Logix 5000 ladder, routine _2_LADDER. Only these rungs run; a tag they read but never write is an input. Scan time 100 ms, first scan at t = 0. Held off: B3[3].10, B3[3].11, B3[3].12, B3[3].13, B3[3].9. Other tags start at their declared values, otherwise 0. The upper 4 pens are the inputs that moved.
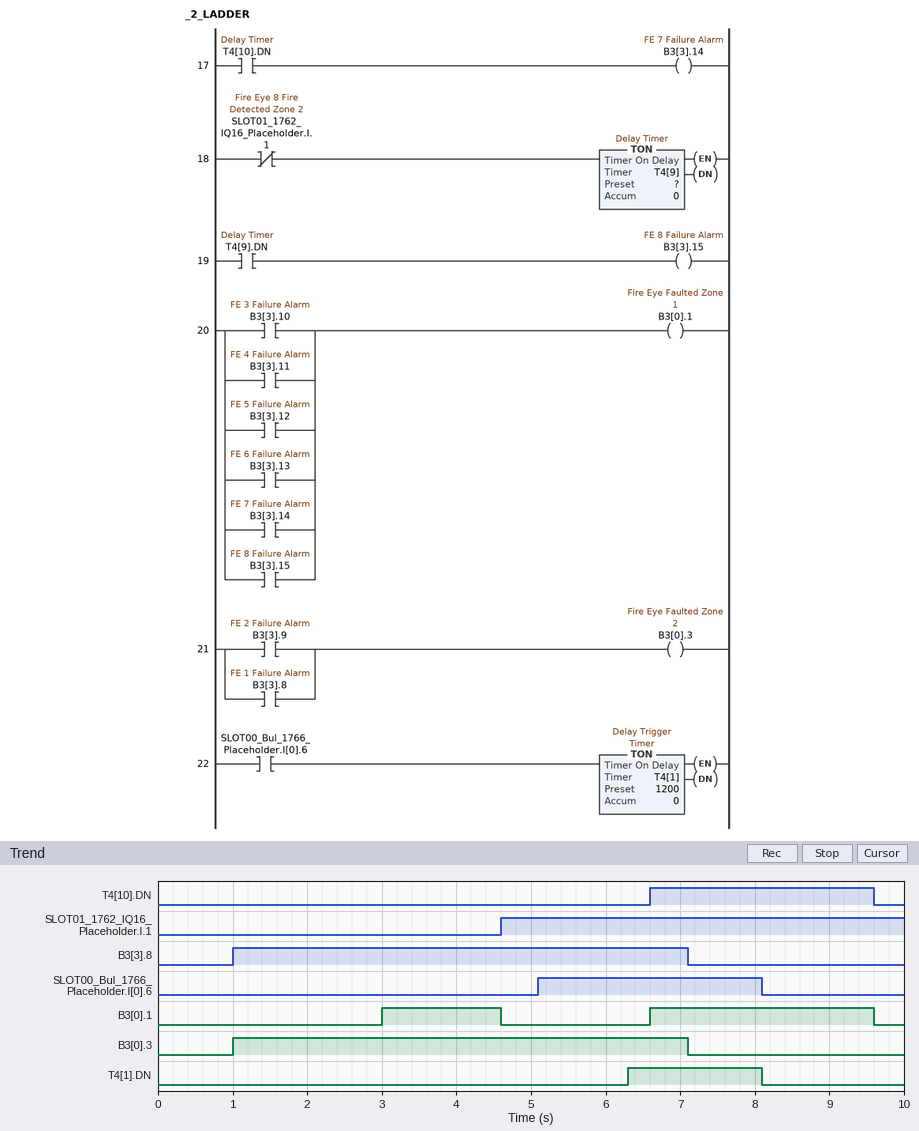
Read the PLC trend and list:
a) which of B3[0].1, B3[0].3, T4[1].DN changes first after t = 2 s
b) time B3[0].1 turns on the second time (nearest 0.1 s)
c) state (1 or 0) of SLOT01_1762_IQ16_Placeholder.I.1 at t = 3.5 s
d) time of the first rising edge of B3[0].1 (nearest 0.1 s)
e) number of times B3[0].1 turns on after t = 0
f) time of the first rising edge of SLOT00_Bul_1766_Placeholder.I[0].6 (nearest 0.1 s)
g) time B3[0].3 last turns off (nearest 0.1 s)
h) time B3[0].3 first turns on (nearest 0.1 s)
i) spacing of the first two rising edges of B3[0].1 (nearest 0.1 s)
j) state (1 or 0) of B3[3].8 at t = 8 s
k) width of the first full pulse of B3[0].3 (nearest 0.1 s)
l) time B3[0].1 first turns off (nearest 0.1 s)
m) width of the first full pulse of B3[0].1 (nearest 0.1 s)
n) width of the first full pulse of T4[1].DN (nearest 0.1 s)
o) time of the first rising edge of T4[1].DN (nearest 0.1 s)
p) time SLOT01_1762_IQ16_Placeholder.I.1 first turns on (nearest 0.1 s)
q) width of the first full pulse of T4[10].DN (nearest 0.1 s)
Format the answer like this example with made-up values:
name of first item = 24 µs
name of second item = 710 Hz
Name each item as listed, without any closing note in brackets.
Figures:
which of B3[0].1, B3[0].3, T4[1].DN changes first after t = 2 s = B3[0].1
time B3[0].1 turns on the second time = 6.6 s
state (1 or 0) of SLOT01_1762_IQ16_Placeholder.I.1 at t = 3.5 s = 0
time of the first rising edge of B3[0].1 = 3.0 s
number of times B3[0].1 turns on after t = 0 = 2
time of the first rising edge of SLOT00_Bul_1766_Placeholder.I[0].6 = 5.1 s
time B3[0].3 last turns off = 7.1 s
time B3[0].3 first turns on = 1.0 s
spacing of the first two rising edges of B3[0].1 = 3.6 s
state (1 or 0) of B3[3].8 at t = 8 s = 0
width of the first full pulse of B3[0].3 = 6.1 s
time B3[0].1 first turns off = 4.6 s
width of the first full pulse of B3[0].1 = 1.6 s
width of the first full pulse of T4[1].DN = 1.8 s
time of the first rising edge of T4[1].DN = 6.3 s
time SLOT01_1762_IQ16_Placeholder.I.1 first turns on = 4.6 s
width of the first full pulse of T4[10].DN = 3.0 s
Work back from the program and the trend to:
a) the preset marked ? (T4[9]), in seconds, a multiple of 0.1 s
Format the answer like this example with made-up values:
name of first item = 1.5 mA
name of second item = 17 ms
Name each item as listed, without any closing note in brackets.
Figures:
the preset marked ? (T4[9]), in seconds, a multiple of 0.1 s = 3.0 s
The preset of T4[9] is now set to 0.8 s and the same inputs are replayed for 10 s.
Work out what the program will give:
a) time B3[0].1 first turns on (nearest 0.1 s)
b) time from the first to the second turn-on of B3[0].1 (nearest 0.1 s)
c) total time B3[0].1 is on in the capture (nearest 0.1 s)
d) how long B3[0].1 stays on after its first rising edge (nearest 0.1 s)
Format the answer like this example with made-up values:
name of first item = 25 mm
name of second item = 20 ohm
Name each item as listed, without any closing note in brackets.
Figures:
time B3[0].1 first turns on = 0.8 s
time from the first to the second turn-on of B3[0].1 = 5.8 s
total time B3[0].1 is on in the capture = 6.8 s
how long B3[0].1 stays on after its first rising edge = 3.8 s
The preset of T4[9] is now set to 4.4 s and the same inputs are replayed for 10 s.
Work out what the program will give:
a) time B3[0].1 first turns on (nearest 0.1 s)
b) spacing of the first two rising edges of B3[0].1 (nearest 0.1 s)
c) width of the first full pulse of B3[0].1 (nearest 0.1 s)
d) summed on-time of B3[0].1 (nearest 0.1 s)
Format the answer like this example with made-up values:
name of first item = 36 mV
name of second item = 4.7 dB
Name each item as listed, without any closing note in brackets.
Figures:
time B3[0].1 first turns on = 4.4 s
spacing of the first two rising edges of B3[0].1 = 2.2 s
width of the first full pulse of B3[0].1 = 0.2 s
summed on-time of B3[0].1 = 3.2 s
